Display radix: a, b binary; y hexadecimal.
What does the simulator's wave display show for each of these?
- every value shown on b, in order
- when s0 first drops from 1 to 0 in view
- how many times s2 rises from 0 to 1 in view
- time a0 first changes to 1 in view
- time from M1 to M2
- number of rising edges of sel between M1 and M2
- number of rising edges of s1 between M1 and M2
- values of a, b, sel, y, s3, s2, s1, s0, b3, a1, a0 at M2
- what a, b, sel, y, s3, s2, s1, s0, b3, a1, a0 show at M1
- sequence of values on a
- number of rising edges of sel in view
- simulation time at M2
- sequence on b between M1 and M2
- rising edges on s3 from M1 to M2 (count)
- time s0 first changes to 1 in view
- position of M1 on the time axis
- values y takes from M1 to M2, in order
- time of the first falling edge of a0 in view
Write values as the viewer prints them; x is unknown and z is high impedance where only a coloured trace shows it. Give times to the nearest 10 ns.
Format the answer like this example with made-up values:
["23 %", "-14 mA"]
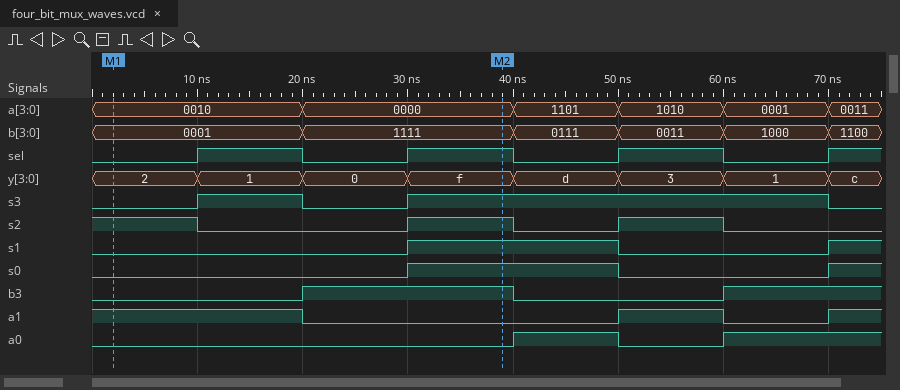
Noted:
["0001, 1111, 0111, 0011, 1000, 1100", "50 ns", "2", "40 ns", "40 ns", "2", "1", "a=0000, b=1111, sel=1, y=f, s3=1, s2=1, s1=1, s0=1, b3=1, a1=0, a0=0", "a=0010, b=0001, sel=0, y=2, s3=0, s2=1, s1=0, s0=0, b3=0, a1=1, a0=0", "0010, 0000, 1101, 1010, 0001, 0011", "4", "40 ns", "0001, 1111", "2", "30 ns", "0 ns", "2, 1, 0, f", "50 ns"]
